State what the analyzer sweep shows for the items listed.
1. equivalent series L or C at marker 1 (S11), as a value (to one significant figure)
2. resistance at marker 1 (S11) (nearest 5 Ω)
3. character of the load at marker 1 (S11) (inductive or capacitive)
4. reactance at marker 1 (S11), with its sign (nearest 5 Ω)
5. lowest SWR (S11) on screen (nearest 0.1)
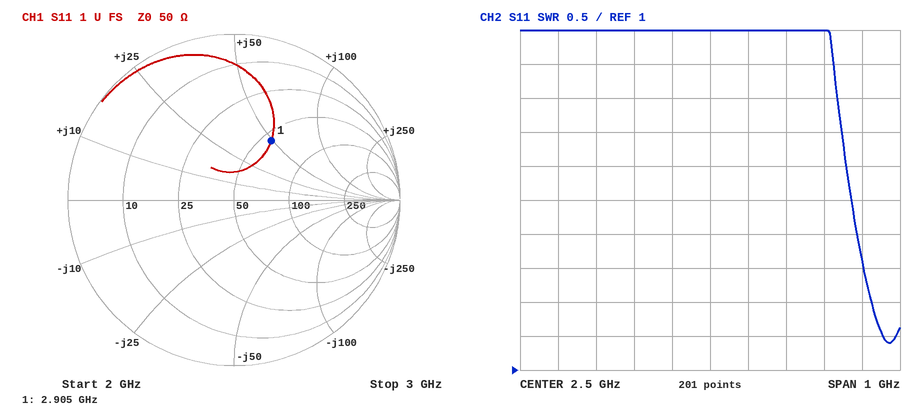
3 nH
55 Ω
inductive
+50 Ω
1.4
